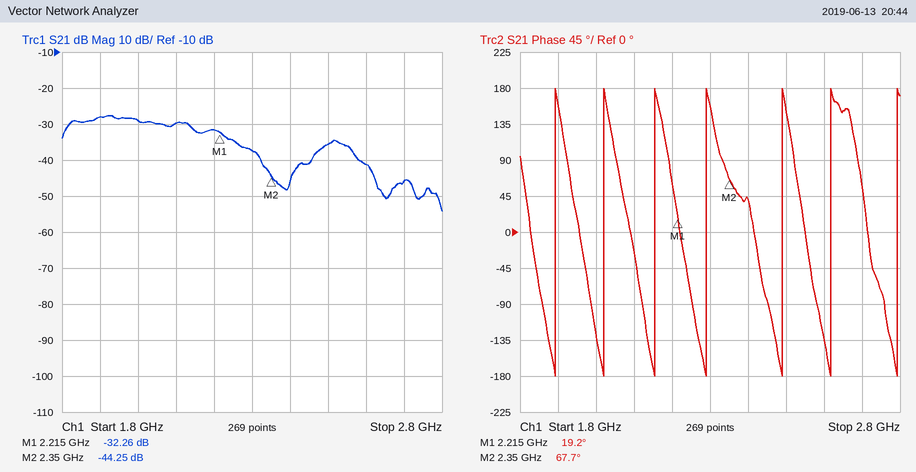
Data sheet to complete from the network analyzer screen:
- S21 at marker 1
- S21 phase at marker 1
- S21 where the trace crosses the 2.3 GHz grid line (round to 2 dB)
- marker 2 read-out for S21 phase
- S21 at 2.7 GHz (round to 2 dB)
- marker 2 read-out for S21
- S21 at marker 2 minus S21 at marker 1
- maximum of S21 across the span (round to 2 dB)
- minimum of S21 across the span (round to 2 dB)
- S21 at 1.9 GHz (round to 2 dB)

-32.26 dB
19.2°
-38 dB
67.7°
-46 dB
-44.25 dB
-11.99 dB
-28 dB
-54 dB
-28 dB
